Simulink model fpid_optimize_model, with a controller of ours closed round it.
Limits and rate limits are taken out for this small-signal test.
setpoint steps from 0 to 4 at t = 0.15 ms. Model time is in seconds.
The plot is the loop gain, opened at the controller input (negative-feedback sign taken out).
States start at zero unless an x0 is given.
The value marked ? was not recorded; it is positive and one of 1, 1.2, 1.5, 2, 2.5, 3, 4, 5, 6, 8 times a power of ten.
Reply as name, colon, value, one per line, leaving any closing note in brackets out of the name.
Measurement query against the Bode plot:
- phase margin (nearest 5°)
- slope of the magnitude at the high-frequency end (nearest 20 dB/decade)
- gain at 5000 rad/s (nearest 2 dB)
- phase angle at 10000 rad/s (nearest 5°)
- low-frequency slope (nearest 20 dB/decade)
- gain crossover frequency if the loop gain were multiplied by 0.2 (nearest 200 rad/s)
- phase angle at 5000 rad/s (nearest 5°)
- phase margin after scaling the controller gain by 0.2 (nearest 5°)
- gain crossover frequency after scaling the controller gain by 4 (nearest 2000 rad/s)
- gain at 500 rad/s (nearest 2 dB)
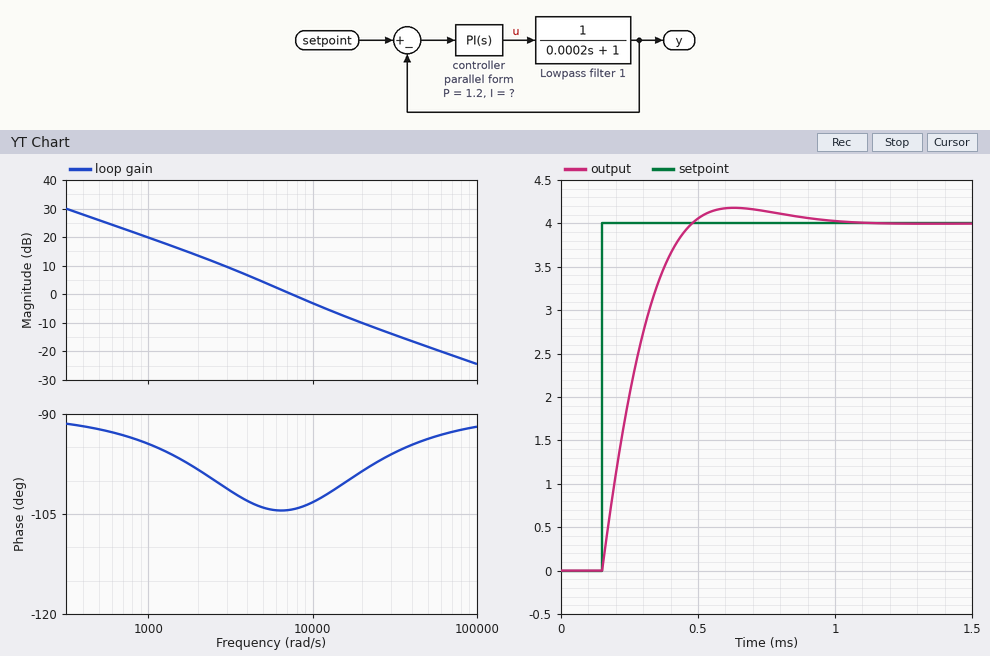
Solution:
phase margin: 75°
slope of the magnitude at the high-frequency end: -20 dB/decade
gain at 5000 rad/s: 4 dB
phase angle at 10000 rad/s: -105°
low-frequency slope: -20 dB/decade
gain crossover frequency if the loop gain were multiplied by 0.2: 2000 rad/s
phase angle at 5000 rad/s: -105°
phase margin after scaling the controller gain by 0.2: 80°
gain crossover frequency after scaling the controller gain by 4: 24000 rad/s
gain at 500 rad/s: 26 dB
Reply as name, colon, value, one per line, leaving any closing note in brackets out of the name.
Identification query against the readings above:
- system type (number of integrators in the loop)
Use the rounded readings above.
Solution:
system type: 1
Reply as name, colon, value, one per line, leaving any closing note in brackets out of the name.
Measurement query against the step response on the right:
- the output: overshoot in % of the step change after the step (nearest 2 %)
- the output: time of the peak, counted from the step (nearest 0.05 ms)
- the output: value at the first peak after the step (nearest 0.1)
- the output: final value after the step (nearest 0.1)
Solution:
the output: overshoot in % of the step change after the step: 4 %
the output: time of the peak, counted from the step: 0.50 ms
the output: value at the first peak after the step: 4.2
the output: final value after the step: 4.0
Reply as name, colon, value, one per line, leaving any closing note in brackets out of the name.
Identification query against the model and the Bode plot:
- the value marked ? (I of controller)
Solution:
the value marked ?: 10000
